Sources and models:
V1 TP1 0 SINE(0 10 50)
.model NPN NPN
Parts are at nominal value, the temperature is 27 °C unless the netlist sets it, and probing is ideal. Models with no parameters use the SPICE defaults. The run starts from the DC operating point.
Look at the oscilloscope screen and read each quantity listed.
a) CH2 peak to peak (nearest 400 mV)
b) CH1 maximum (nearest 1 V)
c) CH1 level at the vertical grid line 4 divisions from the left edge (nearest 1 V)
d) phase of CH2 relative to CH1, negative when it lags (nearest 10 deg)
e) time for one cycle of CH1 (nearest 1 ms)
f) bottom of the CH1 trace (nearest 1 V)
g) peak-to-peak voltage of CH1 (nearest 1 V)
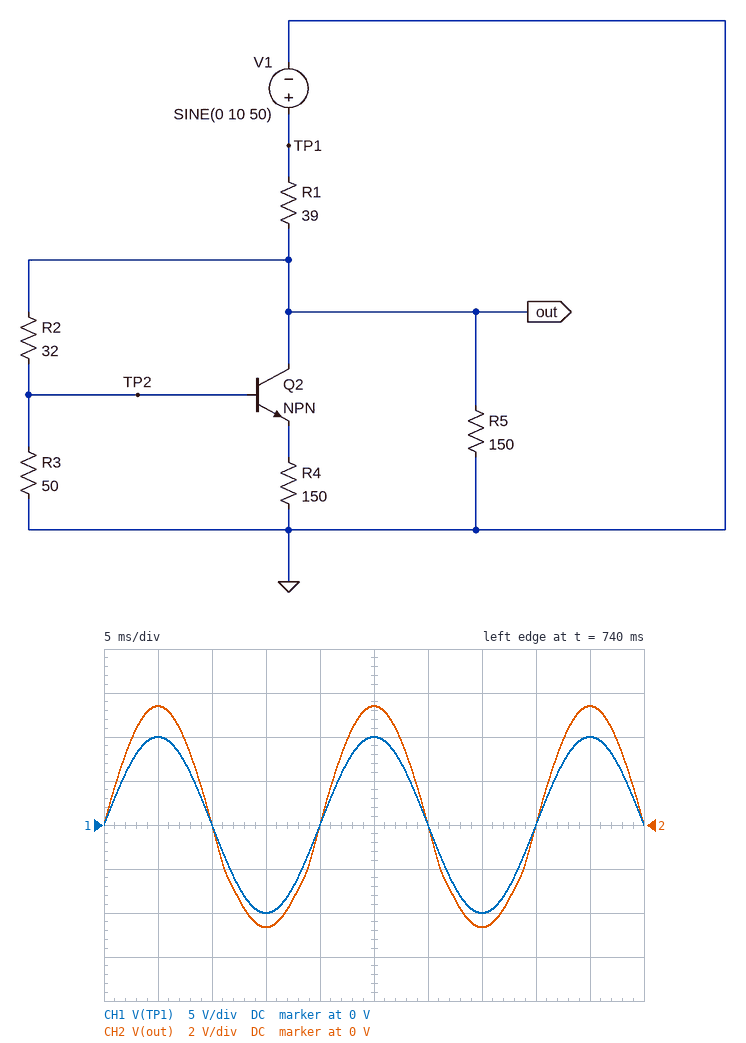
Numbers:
10.0 V
10 V
0 V
0 deg
20 ms
-10 V
20 V
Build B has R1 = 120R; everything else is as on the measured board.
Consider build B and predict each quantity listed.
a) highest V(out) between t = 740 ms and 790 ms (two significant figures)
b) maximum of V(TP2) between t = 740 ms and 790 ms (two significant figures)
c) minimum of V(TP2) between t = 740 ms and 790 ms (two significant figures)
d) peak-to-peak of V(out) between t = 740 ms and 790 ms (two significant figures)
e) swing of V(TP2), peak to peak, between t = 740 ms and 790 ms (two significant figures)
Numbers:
2.8 V
1.7 V
-1.8 V
5.4 V
3.5 V
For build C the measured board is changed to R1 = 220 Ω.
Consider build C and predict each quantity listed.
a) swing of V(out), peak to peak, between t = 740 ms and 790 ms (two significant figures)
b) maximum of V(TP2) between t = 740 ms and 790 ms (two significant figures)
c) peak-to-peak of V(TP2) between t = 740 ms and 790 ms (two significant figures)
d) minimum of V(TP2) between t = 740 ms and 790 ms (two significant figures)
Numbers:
3.8 V
1.1 V
2.3 V
-1.2 V
